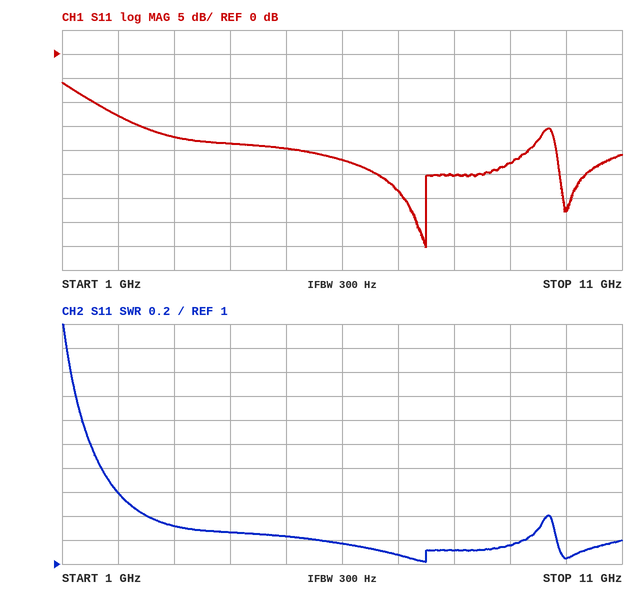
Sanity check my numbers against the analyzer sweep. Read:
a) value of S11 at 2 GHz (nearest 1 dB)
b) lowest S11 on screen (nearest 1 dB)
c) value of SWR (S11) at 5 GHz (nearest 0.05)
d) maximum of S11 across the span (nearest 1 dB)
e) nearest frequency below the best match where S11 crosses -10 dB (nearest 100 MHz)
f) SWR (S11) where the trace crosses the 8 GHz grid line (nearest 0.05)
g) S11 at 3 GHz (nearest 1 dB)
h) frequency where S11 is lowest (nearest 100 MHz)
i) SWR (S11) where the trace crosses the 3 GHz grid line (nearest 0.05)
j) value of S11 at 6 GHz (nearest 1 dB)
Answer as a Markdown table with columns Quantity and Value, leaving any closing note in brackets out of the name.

| Quantity | Value |
|---|---|
| value of S11 at 2 GHz | -13 dB |
| lowest S11 on screen | -40 dB |
| value of SWR (S11) at 5 GHz | 1.25 |
| maximum of S11 across the span | -6 dB |
| nearest frequency below the best match where S11 crosses -10 dB | 1.6 GHz |
| SWR (S11) where the trace crosses the 8 GHz grid line | 1.10 |
| S11 at 3 GHz | -17 dB |
| frequency where S11 is lowest | 7.5 GHz |
| SWR (S11) where the trace crosses the 3 GHz grid line | 1.30 |
| value of S11 at 6 GHz | -22 dB |
